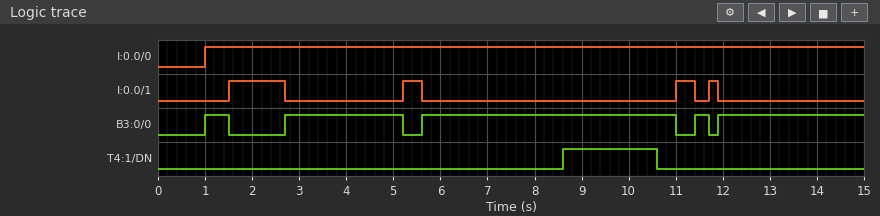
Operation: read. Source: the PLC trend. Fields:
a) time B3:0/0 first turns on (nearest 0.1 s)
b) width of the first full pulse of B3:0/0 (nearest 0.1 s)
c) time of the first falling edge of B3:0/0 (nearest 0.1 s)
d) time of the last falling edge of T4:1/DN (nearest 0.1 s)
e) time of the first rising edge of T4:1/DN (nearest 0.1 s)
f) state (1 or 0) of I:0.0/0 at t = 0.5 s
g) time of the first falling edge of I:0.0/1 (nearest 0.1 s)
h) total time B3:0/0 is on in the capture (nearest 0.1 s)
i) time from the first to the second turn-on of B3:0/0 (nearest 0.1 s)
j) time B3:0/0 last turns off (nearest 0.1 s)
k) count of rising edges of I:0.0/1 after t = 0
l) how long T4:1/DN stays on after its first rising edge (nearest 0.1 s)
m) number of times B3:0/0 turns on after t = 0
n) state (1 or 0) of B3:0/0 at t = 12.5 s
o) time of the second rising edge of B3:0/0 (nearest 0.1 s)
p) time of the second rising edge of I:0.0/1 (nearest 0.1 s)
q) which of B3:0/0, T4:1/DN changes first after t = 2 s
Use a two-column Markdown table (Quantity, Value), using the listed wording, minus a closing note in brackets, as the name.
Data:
| Quantity | Value |
|---|---|
| time B3:0/0 first turns on | 1.0 s |
| width of the first full pulse of B3:0/0 | 0.5 s |
| time of the first falling edge of B3:0/0 | 1.5 s |
| time of the last falling edge of T4:1/DN | 10.6 s |
| time of the first rising edge of T4:1/DN | 8.6 s |
| state (1 or 0) of I:0.0/0 at t = 0.5 s | 0 |
| time of the first falling edge of I:0.0/1 | 2.7 s |
| total time B3:0/0 is on in the capture | 11.8 s |
| time from the first to the second turn-on of B3:0/0 | 1.7 s |
| time B3:0/0 last turns off | 11.7 s |
| count of rising edges of I:0.0/1 after t = 0 | 4 |
| how long T4:1/DN stays on after its first rising edge | 2.0 s |
| number of times B3:0/0 turns on after t = 0 | 5 |
| state (1 or 0) of B3:0/0 at t = 12.5 s | 1 |
| time of the second rising edge of B3:0/0 | 2.7 s |
| time of the second rising edge of I:0.0/1 | 5.2 s |
| which of B3:0/0, T4:1/DN changes first after t = 2 s | B3:0/0 |
